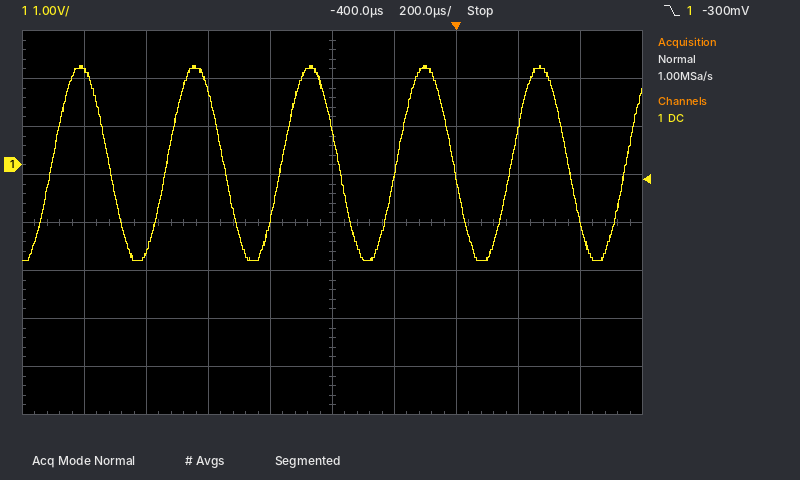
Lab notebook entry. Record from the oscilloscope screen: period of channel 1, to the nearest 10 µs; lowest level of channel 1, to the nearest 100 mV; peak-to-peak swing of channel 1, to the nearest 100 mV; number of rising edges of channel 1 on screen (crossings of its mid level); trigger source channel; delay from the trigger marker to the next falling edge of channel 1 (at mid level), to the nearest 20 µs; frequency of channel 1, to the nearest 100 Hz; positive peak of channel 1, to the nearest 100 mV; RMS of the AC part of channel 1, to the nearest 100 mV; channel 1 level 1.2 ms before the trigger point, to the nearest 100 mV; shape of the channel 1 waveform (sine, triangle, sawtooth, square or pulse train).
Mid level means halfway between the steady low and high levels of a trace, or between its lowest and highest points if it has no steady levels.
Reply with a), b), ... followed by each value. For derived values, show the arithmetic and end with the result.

a) 370 µs
b) -2.0 V
c) 2.1 V − (-2.0 V) = 4.1 V
d) 6
e) channel 1
f) 360 µs
g) 1 / 370 µs ≈ 2.7 kHz
h) 2.1 V
i) 4.1 V / (2√2) ≈ 1.4 V
j) 2.0 V
k) sine
